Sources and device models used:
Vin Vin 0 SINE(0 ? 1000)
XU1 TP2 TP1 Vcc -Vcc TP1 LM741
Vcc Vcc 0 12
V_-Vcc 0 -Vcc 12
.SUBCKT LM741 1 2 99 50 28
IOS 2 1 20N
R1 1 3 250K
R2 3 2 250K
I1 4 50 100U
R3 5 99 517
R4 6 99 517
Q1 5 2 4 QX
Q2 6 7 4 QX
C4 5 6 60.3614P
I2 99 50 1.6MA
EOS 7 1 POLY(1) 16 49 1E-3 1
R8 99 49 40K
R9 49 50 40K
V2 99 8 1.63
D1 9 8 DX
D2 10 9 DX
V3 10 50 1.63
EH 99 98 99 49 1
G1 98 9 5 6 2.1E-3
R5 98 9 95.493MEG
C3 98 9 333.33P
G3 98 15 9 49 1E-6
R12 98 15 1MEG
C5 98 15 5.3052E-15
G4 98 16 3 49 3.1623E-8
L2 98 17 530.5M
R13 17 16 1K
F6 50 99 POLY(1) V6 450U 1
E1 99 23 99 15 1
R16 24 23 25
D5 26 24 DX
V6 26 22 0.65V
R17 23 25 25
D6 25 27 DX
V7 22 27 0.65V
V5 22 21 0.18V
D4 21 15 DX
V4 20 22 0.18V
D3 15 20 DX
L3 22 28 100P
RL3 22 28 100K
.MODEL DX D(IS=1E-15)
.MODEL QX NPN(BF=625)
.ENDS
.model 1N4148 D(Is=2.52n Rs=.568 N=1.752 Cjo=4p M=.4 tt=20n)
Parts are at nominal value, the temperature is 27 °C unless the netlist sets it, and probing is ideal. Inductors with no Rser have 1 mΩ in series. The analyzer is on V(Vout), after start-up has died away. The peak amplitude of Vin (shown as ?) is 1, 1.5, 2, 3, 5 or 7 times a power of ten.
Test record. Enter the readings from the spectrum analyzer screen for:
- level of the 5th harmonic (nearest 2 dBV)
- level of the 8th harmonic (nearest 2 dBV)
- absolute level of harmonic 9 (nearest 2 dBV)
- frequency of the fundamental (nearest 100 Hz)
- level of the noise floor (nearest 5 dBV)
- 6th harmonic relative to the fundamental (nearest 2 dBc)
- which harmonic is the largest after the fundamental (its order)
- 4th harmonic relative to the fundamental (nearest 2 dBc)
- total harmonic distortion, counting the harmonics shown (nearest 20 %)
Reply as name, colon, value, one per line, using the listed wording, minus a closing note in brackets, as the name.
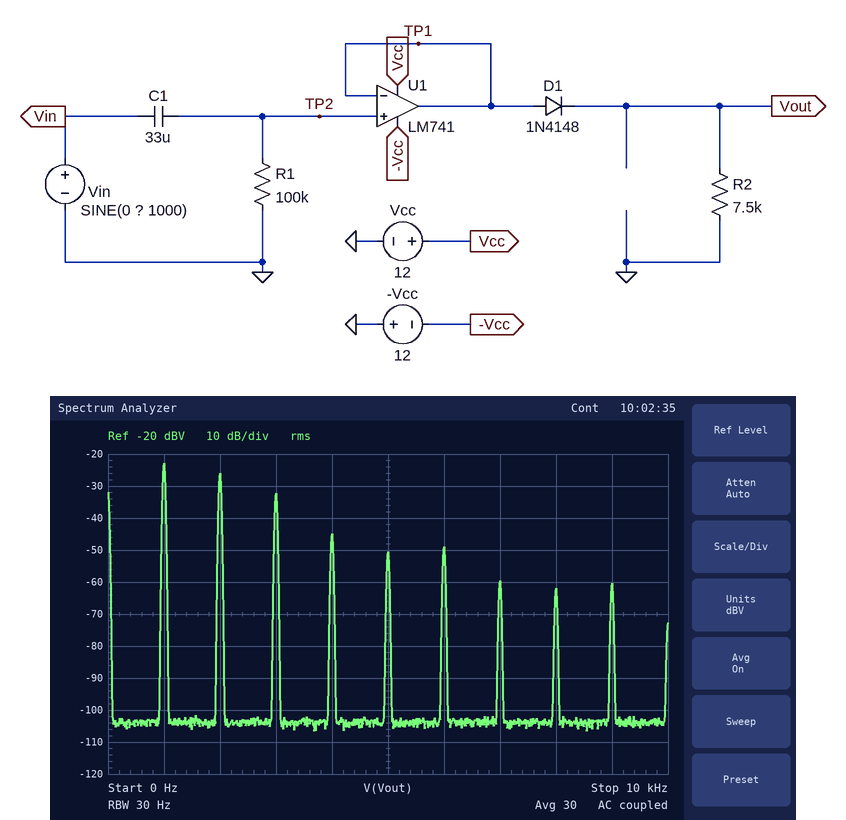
level of the 5th harmonic: -50 dBV
level of the 8th harmonic: -62 dBV
absolute level of harmonic 9: -60 dBV
frequency of the fundamental: 1.0 kHz
level of the noise floor: -105 dBV
6th harmonic relative to the fundamental: -26 dBc
which harmonic is the largest after the fundamental: 2
4th harmonic relative to the fundamental: -22 dBc
total harmonic distortion, counting the harmonics shown: 80 %
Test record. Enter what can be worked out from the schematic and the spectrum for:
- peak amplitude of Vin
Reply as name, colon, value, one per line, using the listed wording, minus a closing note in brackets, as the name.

peak amplitude of Vin: 700 mV
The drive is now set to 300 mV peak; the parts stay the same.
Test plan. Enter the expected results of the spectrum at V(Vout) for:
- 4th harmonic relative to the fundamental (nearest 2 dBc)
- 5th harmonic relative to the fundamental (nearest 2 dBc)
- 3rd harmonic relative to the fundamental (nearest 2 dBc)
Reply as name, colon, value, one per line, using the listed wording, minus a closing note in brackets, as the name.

4th harmonic relative to the fundamental: -12 dBc
5th harmonic relative to the fundamental: -18 dBc
3rd harmonic relative to the fundamental: -6 dBc
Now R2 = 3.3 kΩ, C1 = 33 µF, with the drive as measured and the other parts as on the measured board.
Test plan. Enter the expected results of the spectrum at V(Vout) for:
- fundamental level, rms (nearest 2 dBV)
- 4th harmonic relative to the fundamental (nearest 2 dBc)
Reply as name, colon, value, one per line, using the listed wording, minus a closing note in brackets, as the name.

fundamental level, rms: -24 dBV
4th harmonic relative to the fundamental: -18 dBc
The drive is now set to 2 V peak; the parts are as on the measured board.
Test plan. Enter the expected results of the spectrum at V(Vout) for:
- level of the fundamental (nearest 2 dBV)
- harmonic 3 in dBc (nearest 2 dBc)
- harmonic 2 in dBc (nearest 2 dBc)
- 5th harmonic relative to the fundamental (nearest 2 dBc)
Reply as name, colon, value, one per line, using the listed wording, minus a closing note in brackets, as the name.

level of the fundamental: -6 dBV
harmonic 3 in dBc: -18 dBc
harmonic 2 in dBc: -6 dBc
5th harmonic relative to the fundamental: -26 dBc
